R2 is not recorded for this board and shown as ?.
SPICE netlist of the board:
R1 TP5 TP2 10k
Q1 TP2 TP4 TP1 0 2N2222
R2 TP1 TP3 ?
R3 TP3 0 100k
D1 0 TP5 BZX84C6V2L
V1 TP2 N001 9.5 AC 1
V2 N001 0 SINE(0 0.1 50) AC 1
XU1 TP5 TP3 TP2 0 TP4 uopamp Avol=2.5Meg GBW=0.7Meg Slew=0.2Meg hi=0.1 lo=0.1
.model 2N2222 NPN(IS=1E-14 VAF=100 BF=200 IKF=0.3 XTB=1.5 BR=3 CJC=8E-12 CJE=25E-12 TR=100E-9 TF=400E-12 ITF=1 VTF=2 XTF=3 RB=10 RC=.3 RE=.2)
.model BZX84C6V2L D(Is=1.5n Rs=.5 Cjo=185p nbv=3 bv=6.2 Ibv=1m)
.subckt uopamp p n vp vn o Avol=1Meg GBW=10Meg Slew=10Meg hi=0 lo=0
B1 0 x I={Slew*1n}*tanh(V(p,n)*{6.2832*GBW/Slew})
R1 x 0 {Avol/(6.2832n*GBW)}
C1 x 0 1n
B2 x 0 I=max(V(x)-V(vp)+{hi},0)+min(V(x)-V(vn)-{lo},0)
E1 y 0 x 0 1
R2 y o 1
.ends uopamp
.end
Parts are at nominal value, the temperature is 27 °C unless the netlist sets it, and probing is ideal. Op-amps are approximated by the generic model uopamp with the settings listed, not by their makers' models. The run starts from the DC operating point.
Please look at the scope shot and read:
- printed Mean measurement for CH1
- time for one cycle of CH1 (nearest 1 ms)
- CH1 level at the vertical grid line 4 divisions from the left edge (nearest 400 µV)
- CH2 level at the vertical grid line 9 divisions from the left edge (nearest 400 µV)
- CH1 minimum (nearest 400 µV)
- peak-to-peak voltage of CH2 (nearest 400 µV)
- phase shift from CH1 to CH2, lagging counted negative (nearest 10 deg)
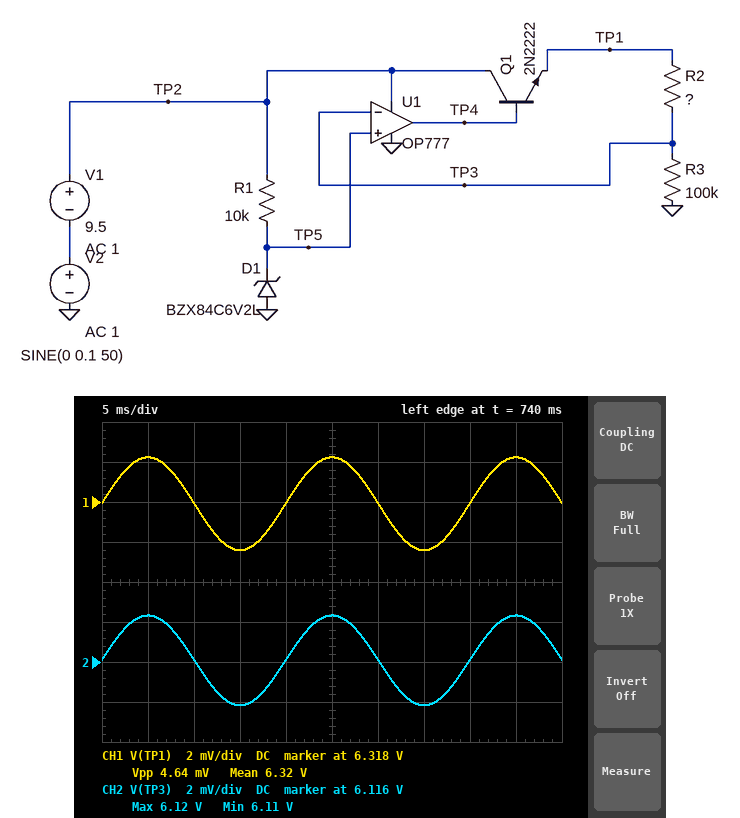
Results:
6.32 V
20 ms
6.3180 V
6.1184 V
6.3156 V
4.4 mV
0 deg
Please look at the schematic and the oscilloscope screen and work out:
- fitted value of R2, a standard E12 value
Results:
3.3 kΩ
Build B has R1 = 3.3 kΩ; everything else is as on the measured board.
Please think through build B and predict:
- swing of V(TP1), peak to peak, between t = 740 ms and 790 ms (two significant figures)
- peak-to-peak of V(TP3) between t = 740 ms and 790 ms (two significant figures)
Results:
4.8 mV
4.6 mV
